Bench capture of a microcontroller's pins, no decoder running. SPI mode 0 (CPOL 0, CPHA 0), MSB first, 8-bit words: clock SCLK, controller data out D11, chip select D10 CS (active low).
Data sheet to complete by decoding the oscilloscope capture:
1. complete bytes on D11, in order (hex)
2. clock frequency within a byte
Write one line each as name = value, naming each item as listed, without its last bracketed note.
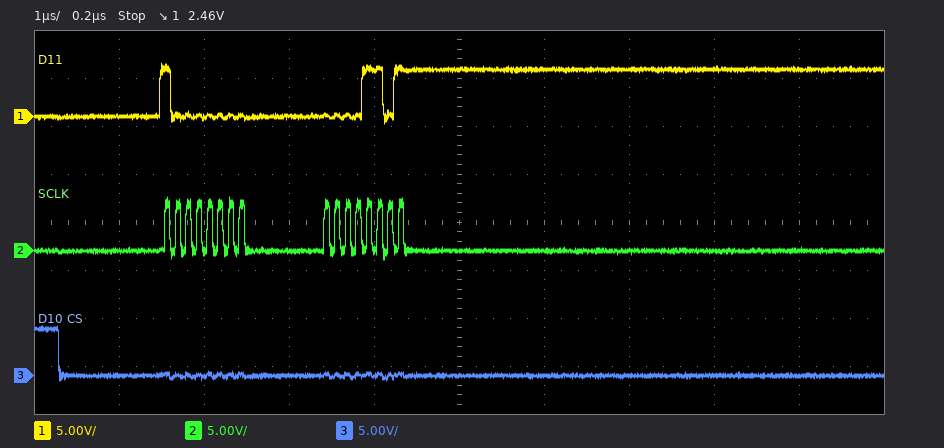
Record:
complete bytes on D11, in order = 80 0D
clock frequency within a byte = 8 MHz
